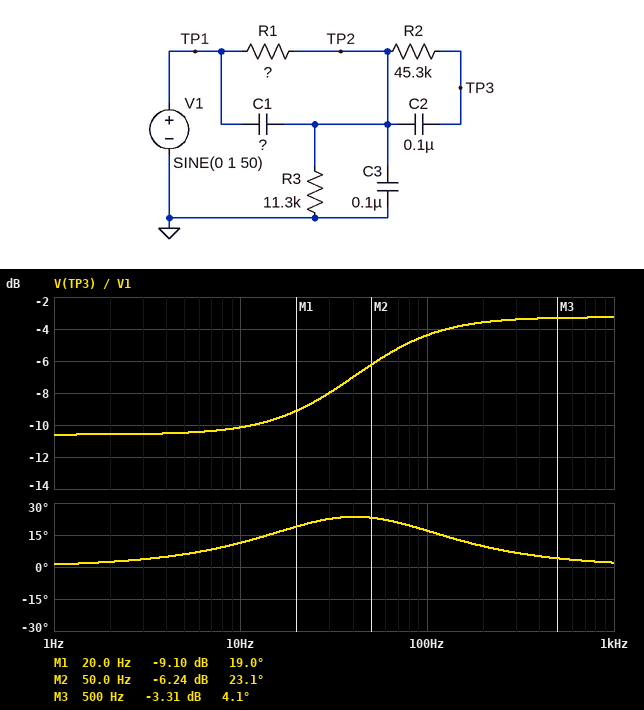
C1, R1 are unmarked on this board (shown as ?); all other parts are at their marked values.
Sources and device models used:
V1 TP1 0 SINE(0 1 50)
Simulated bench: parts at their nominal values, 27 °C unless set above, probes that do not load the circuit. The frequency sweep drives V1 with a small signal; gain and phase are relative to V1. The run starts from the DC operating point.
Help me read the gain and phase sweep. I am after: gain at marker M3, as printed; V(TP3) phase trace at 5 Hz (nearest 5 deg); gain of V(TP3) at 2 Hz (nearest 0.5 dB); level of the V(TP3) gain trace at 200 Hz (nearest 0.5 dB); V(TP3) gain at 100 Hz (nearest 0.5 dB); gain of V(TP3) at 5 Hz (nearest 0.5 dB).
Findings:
-3.31 dB
5 deg
-10.5 dB
-3.5 dB
-4.5 dB
-10.5 dB
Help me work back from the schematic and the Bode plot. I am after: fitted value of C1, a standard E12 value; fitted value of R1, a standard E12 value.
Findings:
220 nF
27 kΩ
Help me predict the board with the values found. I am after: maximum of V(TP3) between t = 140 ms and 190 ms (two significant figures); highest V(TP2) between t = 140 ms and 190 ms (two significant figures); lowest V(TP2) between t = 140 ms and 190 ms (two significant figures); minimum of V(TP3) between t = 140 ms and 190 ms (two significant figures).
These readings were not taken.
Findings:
490 mV
490 mV
-490 mV
-490 mV
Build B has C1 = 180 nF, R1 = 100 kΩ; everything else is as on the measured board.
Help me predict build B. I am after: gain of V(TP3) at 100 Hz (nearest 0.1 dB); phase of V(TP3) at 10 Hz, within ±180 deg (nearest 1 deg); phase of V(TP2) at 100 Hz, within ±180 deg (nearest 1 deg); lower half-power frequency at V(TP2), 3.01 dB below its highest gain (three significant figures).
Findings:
-5.0 dB
38 deg
24 deg
54.6 Hz
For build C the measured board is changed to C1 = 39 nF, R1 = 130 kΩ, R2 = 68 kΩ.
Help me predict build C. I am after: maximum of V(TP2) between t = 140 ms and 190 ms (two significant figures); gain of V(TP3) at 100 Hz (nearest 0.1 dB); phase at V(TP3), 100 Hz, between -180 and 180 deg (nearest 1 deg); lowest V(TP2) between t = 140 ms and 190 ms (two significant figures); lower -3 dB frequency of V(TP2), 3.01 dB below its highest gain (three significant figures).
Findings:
140 mV
-14.1 dB
30 deg
-140 mV
101 Hz
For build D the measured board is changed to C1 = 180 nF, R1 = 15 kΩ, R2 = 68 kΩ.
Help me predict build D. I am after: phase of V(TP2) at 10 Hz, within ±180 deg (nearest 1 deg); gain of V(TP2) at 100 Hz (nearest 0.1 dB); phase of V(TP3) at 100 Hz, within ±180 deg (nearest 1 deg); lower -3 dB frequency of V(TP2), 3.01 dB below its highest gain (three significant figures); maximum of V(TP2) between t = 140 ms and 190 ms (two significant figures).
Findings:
3 deg
-5.0 dB
11 deg
28.8 Hz
490 mV
